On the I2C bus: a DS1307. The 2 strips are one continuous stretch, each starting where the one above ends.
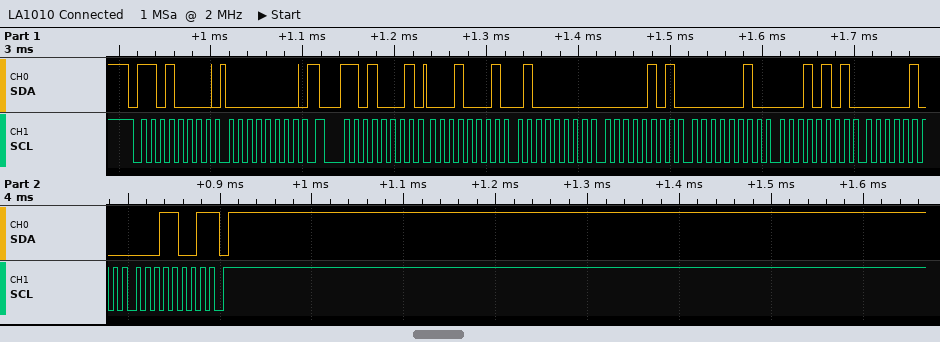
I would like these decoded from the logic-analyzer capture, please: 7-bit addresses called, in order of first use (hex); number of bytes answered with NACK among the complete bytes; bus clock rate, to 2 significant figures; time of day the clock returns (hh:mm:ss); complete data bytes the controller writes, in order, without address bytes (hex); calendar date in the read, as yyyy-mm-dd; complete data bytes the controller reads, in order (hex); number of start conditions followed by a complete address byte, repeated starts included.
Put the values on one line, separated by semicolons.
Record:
0x68; 1; 100 kHz; 05:40:11; 00; 2019-04-15; 11 40 05 02 15 04 19; 2
